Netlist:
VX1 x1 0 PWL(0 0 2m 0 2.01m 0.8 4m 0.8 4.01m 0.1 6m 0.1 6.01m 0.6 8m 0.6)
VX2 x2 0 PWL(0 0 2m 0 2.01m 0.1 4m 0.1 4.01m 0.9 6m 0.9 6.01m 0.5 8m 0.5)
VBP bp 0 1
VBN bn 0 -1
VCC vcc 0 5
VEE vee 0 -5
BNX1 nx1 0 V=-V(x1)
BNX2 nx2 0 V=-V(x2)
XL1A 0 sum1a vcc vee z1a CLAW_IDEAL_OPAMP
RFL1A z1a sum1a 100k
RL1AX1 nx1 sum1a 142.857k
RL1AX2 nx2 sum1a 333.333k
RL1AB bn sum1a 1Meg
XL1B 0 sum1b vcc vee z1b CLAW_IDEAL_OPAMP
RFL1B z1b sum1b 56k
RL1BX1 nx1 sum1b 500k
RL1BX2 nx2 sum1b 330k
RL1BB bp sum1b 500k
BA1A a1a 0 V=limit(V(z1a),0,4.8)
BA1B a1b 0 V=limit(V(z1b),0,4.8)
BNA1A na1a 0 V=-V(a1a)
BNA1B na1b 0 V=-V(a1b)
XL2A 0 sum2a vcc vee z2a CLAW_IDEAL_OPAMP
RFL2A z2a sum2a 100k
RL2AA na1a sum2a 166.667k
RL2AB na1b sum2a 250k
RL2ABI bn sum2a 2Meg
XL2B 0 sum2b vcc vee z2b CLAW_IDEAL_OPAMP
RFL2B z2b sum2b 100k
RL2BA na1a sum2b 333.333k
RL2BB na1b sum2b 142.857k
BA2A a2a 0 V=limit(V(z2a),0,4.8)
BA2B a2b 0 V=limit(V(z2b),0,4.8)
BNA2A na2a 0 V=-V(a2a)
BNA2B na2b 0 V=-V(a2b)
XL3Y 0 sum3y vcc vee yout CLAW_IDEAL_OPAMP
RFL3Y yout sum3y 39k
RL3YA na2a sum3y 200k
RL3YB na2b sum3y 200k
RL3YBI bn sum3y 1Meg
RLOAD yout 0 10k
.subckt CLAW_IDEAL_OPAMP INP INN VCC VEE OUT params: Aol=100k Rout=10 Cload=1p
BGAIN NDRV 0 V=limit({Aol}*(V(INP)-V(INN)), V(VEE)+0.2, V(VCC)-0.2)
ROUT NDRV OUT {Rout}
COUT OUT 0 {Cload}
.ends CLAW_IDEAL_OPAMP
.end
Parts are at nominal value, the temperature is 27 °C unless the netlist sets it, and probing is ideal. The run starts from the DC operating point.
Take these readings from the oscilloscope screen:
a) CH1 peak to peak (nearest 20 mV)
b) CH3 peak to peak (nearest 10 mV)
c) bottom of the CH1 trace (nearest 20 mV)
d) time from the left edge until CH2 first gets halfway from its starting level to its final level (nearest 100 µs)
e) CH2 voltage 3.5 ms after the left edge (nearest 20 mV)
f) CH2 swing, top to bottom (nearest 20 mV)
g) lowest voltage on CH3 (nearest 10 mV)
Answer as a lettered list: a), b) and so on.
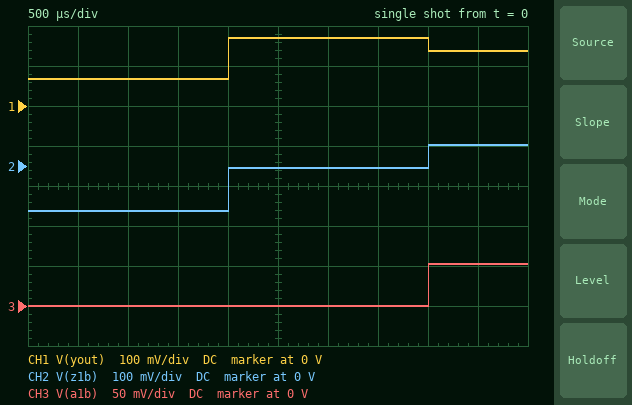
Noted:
a) 100 mV
b) 50 mV
c) 60 mV
d) 2.0 ms
e) 0 V
f) 160 mV
g) 0 V
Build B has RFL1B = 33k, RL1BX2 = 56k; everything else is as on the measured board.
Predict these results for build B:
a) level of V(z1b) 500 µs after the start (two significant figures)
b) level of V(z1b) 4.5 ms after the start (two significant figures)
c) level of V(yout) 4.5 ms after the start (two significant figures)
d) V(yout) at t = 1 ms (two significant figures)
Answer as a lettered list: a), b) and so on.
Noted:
a) -66 mV
b) 470 mV
c) 230 mV
d) 66 mV
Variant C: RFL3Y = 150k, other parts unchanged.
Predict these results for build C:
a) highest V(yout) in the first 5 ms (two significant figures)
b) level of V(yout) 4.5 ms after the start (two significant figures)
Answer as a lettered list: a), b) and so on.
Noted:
a) 650 mV
b) 530 mV
